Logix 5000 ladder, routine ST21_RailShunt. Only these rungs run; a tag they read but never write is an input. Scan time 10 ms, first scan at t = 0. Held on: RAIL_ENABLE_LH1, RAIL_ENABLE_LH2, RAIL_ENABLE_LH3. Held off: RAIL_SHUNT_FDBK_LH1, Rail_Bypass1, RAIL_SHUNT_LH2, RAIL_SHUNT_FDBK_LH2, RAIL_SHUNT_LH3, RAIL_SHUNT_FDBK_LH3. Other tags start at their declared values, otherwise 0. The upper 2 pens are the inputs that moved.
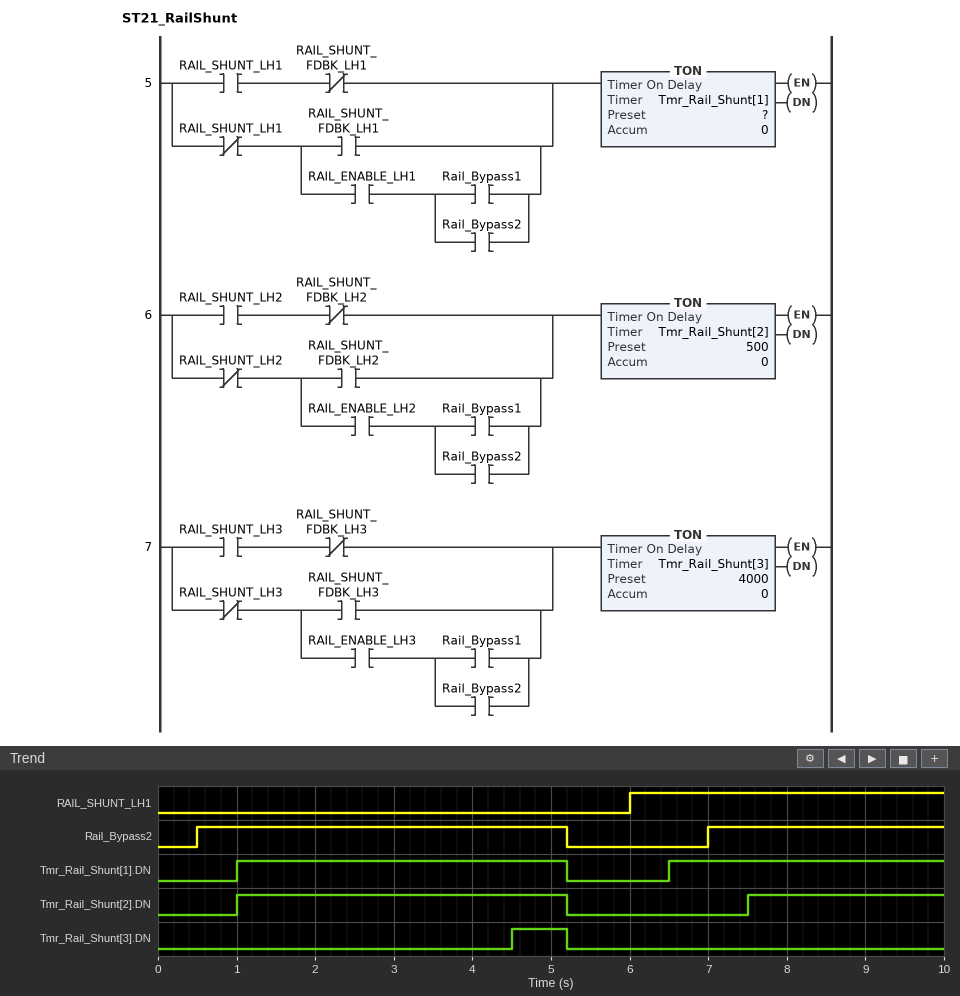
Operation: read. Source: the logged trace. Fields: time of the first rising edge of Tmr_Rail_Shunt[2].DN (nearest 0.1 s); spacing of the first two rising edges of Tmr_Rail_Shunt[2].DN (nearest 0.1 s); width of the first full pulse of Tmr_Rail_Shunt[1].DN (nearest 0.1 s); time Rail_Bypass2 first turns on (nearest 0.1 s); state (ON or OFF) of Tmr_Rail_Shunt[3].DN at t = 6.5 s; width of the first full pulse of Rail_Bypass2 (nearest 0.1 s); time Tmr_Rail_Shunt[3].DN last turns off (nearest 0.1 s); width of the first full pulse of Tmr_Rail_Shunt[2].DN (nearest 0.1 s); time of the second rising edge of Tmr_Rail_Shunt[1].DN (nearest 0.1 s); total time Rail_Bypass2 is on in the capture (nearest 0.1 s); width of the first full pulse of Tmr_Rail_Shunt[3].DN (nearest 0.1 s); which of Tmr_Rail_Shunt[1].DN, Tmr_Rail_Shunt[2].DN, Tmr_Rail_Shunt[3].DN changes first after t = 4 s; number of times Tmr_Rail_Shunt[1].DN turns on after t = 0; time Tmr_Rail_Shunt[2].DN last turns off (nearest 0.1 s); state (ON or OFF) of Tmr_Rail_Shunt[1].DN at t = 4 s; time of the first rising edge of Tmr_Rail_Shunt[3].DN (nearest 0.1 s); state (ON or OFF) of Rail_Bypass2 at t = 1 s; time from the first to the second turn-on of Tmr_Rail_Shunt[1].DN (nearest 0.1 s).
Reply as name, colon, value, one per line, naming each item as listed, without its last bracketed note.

time of the first rising edge of Tmr_Rail_Shunt[2].DN: 1.0 s
spacing of the first two rising edges of Tmr_Rail_Shunt[2].DN: 6.5 s
width of the first full pulse of Tmr_Rail_Shunt[1].DN: 4.2 s
time Rail_Bypass2 first turns on: 0.5 s
state (ON or OFF) of Tmr_Rail_Shunt[3].DN at t = 6.5 s: OFF
width of the first full pulse of Rail_Bypass2: 4.7 s
time Tmr_Rail_Shunt[3].DN last turns off: 5.2 s
width of the first full pulse of Tmr_Rail_Shunt[2].DN: 4.2 s
time of the second rising edge of Tmr_Rail_Shunt[1].DN: 6.5 s
total time Rail_Bypass2 is on in the capture: 7.7 s
width of the first full pulse of Tmr_Rail_Shunt[3].DN: 0.7 s
which of Tmr_Rail_Shunt[1].DN, Tmr_Rail_Shunt[2].DN, Tmr_Rail_Shunt[3].DN changes first after t = 4 s: Tmr_Rail_Shunt[3].DN
number of times Tmr_Rail_Shunt[1].DN turns on after t = 0: 2
time Tmr_Rail_Shunt[2].DN last turns off: 5.2 s
state (ON or OFF) of Tmr_Rail_Shunt[1].DN at t = 4 s: ON
time of the first rising edge of Tmr_Rail_Shunt[3].DN: 4.5 s
state (ON or OFF) of Rail_Bypass2 at t = 1 s: ON
time from the first to the second turn-on of Tmr_Rail_Shunt[1].DN: 5.5 s
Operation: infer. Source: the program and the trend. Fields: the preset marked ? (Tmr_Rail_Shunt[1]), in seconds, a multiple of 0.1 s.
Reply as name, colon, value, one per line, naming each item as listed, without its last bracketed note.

the preset marked ? (Tmr_Rail_Shunt[1]), in seconds, a multiple of 0.1 s: 0.5 s
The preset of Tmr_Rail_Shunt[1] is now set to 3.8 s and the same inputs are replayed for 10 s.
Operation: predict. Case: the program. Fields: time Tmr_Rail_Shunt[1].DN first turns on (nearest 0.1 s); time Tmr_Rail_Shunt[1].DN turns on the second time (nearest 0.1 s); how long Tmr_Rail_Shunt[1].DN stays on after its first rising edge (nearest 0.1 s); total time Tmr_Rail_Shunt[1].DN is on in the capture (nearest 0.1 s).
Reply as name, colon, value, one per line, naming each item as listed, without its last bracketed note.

time Tmr_Rail_Shunt[1].DN first turns on: 4.3 s
time Tmr_Rail_Shunt[1].DN turns on the second time: 9.8 s
how long Tmr_Rail_Shunt[1].DN stays on after its first rising edge: 0.9 s
total time Tmr_Rail_Shunt[1].DN is on in the capture: 1.1 s
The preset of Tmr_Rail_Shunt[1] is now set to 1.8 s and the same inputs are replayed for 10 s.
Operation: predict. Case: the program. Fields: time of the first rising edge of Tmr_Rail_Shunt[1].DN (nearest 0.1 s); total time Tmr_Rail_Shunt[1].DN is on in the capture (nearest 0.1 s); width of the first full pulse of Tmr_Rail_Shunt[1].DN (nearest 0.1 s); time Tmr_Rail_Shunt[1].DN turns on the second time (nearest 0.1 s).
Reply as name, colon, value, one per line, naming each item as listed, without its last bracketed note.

time of the first rising edge of Tmr_Rail_Shunt[1].DN: 2.3 s
total time Tmr_Rail_Shunt[1].DN is on in the capture: 5.1 s
width of the first full pulse of Tmr_Rail_Shunt[1].DN: 2.9 s
time Tmr_Rail_Shunt[1].DN turns on the second time: 7.8 s
